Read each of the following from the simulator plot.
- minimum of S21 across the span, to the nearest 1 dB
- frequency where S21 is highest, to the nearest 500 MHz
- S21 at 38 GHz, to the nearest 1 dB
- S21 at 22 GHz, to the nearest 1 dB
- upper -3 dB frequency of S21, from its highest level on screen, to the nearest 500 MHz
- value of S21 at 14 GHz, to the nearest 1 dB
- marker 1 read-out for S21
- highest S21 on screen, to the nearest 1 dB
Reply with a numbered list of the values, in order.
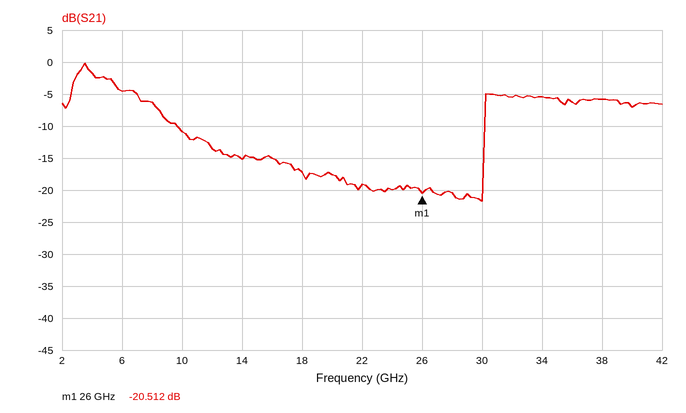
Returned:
1. -22 dB
2. 3.5 GHz
3. -6 dB
4. -19 dB
5. 5.5 GHz
6. -15 dB
7. -20.512 dB
8. 0 dB
